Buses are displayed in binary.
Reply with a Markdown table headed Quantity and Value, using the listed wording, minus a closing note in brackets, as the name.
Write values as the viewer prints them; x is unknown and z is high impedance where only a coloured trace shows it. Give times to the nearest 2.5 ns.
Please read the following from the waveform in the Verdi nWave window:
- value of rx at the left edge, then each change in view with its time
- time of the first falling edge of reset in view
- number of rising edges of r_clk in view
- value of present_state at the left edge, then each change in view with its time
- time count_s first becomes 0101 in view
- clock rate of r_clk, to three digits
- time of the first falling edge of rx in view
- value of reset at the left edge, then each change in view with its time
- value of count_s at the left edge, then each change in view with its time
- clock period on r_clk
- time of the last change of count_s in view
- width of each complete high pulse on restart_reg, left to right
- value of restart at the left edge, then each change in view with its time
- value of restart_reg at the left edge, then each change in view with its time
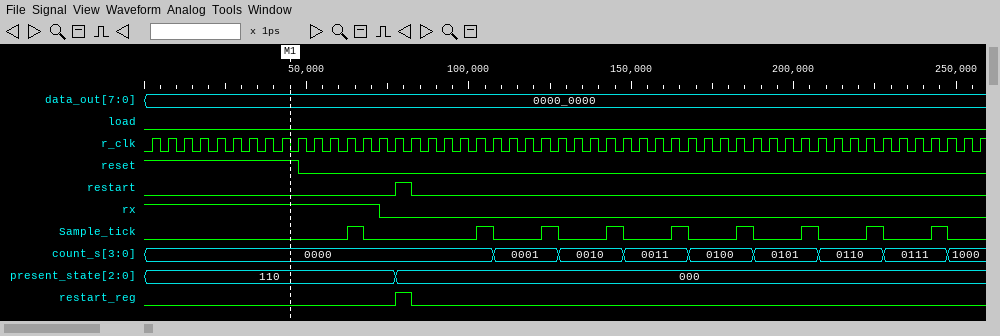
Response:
| Quantity | Value |
|---|---|
| value of rx at the left edge, then each change in view with its time | 1, 0 at 72.5 ns |
| time of the first falling edge of reset in view | 47.5 ns |
| number of rising edges of r_clk in view | 52 |
| value of present_state at the left edge, then each change in view with its time | 110, 000 at 77.5 ns |
| time count_s first becomes 0101 in view | 187.5 ns |
| clock rate of r_clk, to three digits | 200 MHz |
| time of the first falling edge of rx in view | 72.5 ns |
| value of reset at the left edge, then each change in view with its time | 1, 0 at 47.5 ns |
| value of count_s at the left edge, then each change in view with its time | 0000, 0001 at 107.5 ns, 0010 at 127.5 ns, 0011 at 147.5 ns, 0100 at 167.5 ns, 0101 at 187.5 ns, 0110 at 207.5 ns, 0111 at 227.5 ns, 1000 at 247.5 ns |
| clock period on r_clk | 5 ns |
| time of the last change of count_s in view | 247.5 ns |
| width of each complete high pulse on restart_reg, left to right | 5 ns |
| value of restart at the left edge, then each change in view with its time | 0, 1 at 77.5 ns, 0 at 82.5 ns |
| value of restart_reg at the left edge, then each change in view with its time | 0, 1 at 77.5 ns, 0 at 82.5 ns |
